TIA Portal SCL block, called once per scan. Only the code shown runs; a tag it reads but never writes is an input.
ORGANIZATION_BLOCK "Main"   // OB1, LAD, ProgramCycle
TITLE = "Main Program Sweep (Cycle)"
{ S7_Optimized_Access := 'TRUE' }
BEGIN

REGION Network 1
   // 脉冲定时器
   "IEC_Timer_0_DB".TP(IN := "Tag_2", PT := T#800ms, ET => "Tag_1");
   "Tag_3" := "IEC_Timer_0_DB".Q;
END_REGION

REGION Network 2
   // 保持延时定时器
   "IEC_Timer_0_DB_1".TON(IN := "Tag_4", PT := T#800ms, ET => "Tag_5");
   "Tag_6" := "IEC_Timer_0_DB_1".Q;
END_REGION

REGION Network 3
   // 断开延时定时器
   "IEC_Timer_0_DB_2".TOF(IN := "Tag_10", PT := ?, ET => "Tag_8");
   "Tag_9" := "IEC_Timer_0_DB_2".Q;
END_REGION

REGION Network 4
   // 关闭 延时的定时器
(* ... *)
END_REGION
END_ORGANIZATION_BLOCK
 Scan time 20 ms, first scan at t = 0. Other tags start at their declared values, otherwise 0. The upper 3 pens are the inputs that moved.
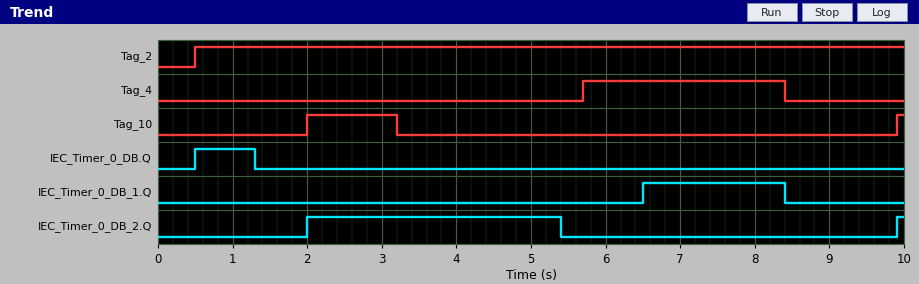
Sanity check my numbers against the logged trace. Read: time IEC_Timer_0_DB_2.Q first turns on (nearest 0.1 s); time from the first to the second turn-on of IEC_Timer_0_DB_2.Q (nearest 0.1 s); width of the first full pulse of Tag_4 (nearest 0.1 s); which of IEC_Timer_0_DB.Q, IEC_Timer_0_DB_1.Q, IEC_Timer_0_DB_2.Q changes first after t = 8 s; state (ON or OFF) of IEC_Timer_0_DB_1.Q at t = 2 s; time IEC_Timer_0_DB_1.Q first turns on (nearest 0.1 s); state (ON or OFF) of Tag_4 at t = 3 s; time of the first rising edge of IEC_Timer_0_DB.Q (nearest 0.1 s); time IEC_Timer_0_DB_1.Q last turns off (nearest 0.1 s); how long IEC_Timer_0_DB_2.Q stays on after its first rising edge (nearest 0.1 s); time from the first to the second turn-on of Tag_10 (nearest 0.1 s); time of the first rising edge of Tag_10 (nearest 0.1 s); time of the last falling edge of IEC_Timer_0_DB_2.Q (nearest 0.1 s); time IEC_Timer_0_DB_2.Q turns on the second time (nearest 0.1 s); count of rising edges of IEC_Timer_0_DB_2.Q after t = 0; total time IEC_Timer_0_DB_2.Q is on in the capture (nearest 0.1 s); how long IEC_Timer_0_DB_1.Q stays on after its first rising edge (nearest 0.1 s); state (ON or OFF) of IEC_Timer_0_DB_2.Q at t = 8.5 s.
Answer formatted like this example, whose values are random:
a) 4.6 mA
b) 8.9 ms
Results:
a) 2.0 s
b) 7.9 s
c) 2.7 s
d) IEC_Timer_0_DB_1.Q
e) OFF
f) 6.5 s
g) OFF
h) 0.5 s
i) 8.4 s
j) 3.4 s
k) 7.9 s
l) 2.0 s
m) 5.4 s
n) 9.9 s
o) 2
p) 3.5 s
q) 1.9 s
r) OFF
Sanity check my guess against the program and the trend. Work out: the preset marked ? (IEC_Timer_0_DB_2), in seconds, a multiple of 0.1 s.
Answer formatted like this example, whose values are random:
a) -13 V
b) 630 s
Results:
a) 2.2 s
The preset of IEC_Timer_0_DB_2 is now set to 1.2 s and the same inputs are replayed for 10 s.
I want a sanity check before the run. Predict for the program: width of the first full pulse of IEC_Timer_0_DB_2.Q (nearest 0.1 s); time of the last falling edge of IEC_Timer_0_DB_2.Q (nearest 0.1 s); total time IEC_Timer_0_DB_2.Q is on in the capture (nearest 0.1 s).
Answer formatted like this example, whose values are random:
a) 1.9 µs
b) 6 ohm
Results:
a) 2.4 s
b) 4.4 s
c) 2.5 s
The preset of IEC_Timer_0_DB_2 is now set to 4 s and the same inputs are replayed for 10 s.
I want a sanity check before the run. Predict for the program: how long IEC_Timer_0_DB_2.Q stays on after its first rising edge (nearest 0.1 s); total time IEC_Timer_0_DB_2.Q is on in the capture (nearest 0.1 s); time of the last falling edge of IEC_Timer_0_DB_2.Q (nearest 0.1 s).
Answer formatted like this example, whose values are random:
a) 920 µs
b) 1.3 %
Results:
a) 5.2 s
b) 5.3 s
c) 7.2 s
